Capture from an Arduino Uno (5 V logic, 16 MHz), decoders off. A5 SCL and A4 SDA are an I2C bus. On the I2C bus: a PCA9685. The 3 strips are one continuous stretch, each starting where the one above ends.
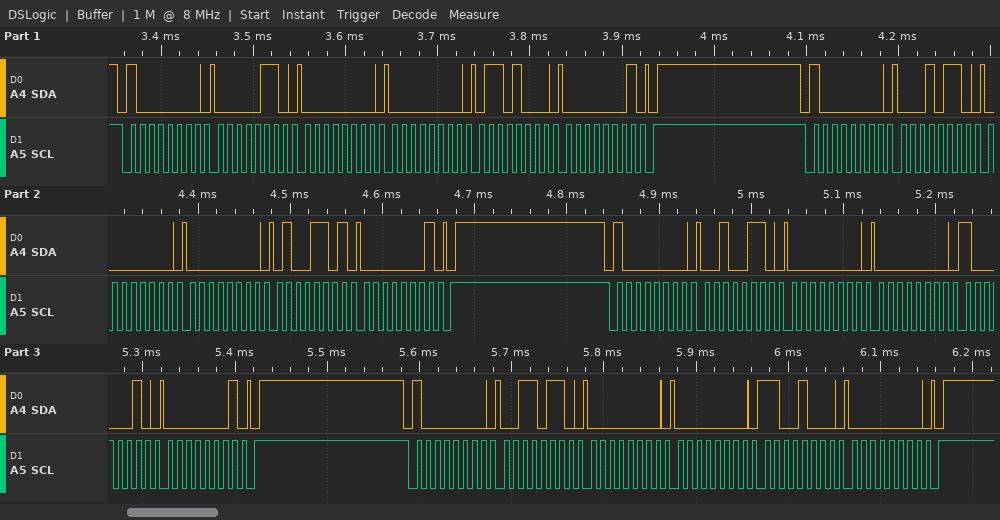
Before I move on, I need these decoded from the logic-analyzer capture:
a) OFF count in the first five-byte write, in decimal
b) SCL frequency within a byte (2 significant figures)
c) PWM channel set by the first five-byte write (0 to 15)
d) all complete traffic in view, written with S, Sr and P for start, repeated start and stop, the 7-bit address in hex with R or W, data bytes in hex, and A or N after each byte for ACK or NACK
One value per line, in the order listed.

360
100 kHz
0
S 40W A 06 A 00 A 00 A 68 A 01 A P S 40W A 16 A 00 A 00 A 4D A 01 A P S 40W A 26 A 00 A 00 A 82 A 01 A P S 40W A 36 A 00 A 00 A C8 A 00 A P
